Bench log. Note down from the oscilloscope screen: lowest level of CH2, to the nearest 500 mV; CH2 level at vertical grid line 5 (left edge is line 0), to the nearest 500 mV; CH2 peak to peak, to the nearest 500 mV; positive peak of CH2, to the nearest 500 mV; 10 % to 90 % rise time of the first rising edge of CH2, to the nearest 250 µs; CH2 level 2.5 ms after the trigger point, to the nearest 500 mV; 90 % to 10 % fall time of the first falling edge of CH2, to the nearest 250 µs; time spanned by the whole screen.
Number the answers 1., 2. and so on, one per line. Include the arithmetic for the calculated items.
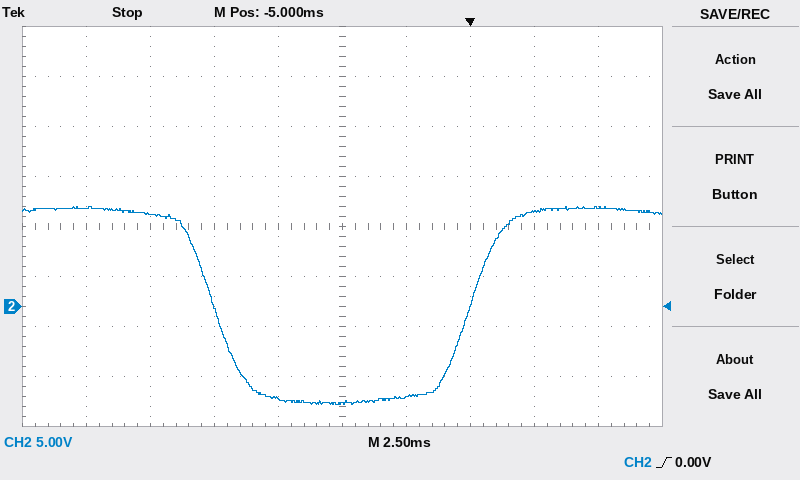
1. -10.0 V
2. -9.5 V
3. 10.0 V − (-10.0 V) = 20.0 V
4. 10.0 V
5. 2.50 ms
6. 9.5 V
7. 2.50 ms
8. 25 ms
